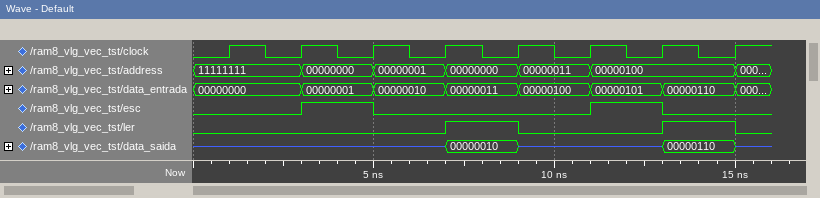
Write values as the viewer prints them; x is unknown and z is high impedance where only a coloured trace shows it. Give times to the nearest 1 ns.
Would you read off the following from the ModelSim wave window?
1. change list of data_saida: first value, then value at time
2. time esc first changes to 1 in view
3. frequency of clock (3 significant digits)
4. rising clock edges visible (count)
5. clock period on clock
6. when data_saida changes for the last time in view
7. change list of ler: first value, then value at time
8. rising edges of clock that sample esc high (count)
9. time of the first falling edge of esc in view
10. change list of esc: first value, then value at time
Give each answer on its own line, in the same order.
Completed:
z, 00000010 at 7 ns, z at 9 ns, 00000110 at 13 ns, z at 15 ns
3 ns
500 MHz
8
2 ns
15 ns
0, 1 at 7 ns, 0 at 9 ns, 1 at 13 ns, 0 at 15 ns
2
5 ns
0, 1 at 3 ns, 0 at 5 ns, 1 at 11 ns, 0 at 13 ns
